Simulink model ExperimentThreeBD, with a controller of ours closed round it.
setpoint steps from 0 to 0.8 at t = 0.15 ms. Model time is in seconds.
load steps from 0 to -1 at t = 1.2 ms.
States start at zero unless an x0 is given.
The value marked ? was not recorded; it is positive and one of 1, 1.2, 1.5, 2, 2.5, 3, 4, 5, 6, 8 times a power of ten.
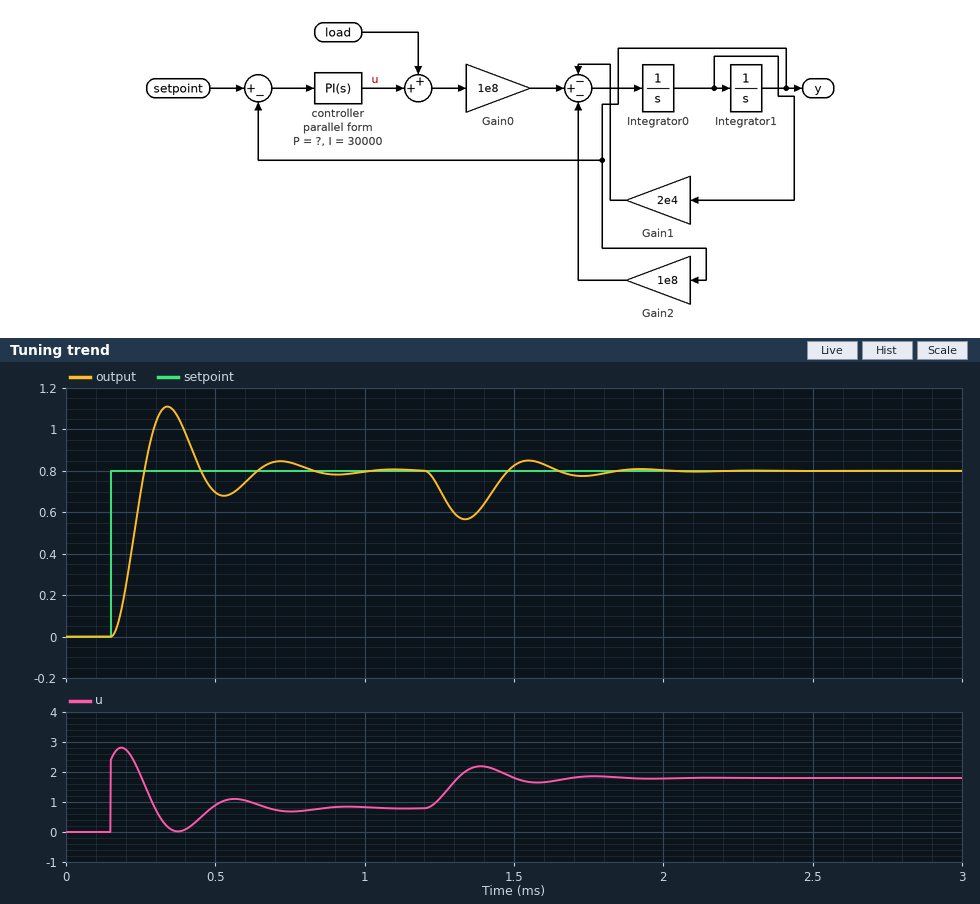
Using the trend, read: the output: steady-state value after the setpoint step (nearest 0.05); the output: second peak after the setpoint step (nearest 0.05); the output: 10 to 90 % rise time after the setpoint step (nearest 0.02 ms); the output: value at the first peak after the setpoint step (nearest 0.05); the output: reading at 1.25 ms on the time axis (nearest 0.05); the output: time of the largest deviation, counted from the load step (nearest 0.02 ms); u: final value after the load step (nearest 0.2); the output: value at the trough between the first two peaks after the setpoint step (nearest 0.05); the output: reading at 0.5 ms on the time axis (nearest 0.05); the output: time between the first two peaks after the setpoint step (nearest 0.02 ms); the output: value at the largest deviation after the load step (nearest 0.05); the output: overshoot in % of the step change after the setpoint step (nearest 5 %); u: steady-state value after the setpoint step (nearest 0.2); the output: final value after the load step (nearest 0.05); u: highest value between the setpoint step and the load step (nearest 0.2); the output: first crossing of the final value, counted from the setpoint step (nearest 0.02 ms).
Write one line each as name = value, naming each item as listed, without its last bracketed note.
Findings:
the output: steady-state value after the setpoint step = 0.80
the output: second peak after the setpoint step = 0.85
the output: 10 to 90 % rise time after the setpoint step = 0.08 ms
the output: value at the first peak after the setpoint step = 1.10
the output: reading at 1.25 ms on the time axis = 0.70
the output: time of the largest deviation, counted from the load step = 0.14 ms
u: final value after the load step = 1.8
the output: value at the trough between the first two peaks after the setpoint step = 0.70
the output: reading at 0.5 ms on the time axis = 0.70
the output: time between the first two peaks after the setpoint step = 0.38 ms
the output: value at the largest deviation after the load step = 0.55
the output: overshoot in % of the step change after the setpoint step = 40 %
u: steady-state value after the setpoint step = 0.8
the output: final value after the load step = 0.80
u: highest value between the setpoint step and the load step = 2.8
the output: first crossing of the final value, counted from the setpoint step = 0.12 ms
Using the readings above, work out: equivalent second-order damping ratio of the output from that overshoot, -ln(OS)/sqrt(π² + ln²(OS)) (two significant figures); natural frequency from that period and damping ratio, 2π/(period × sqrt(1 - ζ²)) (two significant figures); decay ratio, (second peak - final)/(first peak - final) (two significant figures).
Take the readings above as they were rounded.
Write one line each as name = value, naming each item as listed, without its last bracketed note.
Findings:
equivalent second-order damping ratio of the output from that overshoot, -ln(OS)/sqrt(π² + ln²(OS)) = 0.28
natural frequency from that period and damping ratio, 2π/(period × sqrt(1 - ζ²)) = 17 rad/ms
decay ratio, (second peak - final)/(first peak - final) = 0.17
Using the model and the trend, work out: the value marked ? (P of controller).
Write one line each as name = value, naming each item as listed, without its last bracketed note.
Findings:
the value marked ? = 3
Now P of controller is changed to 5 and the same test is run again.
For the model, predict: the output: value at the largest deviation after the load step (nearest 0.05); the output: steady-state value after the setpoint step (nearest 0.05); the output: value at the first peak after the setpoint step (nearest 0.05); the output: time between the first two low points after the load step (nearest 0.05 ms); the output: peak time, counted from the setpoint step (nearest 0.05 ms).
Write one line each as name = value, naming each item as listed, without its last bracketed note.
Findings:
the output: value at the largest deviation after the load step = 0.60
the output: steady-state value after the setpoint step = 0.80
the output: value at the first peak after the setpoint step = 1.05
the output: time between the first two low points after the load step = 0.30 ms
the output: peak time, counted from the setpoint step = 0.15 ms
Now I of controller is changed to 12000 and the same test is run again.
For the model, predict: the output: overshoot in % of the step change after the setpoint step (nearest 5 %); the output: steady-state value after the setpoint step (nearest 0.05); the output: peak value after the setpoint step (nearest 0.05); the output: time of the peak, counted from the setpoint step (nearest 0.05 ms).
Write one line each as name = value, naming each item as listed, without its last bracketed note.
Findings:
the output: overshoot in % of the step change after the setpoint step = 10 %
the output: steady-state value after the setpoint step = 0.80
the output: peak value after the setpoint step = 0.90
the output: time of the peak, counted from the setpoint step = 0.20 ms
